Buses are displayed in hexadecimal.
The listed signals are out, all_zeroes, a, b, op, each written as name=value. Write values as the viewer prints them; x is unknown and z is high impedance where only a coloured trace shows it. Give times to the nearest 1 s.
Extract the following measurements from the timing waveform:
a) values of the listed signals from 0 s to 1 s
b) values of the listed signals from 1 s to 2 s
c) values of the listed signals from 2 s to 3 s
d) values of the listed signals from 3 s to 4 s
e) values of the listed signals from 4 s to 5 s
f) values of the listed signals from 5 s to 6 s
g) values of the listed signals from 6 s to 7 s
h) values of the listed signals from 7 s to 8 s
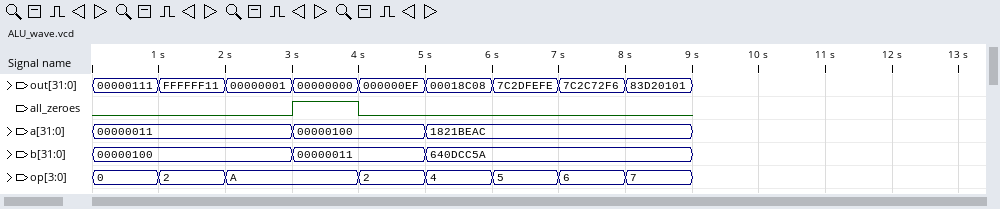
out=00000111, all_zeroes=0, a=00000011, b=00000100, op=0
out=FFFFFF11, all_zeroes=0, a=00000011, b=00000100, op=2
out=00000001, all_zeroes=0, a=00000011, b=00000100, op=A
out=00000000, all_zeroes=1, a=00000100, b=00000011, op=A
out=000000EF, all_zeroes=0, a=00000100, b=00000011, op=2
out=00018C08, all_zeroes=0, a=1821BEAC, b=640DCC5A, op=4
out=7C2DFEFE, all_zeroes=0, a=1821BEAC, b=640DCC5A, op=5
out=7C2C72F6, all_zeroes=0, a=1821BEAC, b=640DCC5A, op=6
